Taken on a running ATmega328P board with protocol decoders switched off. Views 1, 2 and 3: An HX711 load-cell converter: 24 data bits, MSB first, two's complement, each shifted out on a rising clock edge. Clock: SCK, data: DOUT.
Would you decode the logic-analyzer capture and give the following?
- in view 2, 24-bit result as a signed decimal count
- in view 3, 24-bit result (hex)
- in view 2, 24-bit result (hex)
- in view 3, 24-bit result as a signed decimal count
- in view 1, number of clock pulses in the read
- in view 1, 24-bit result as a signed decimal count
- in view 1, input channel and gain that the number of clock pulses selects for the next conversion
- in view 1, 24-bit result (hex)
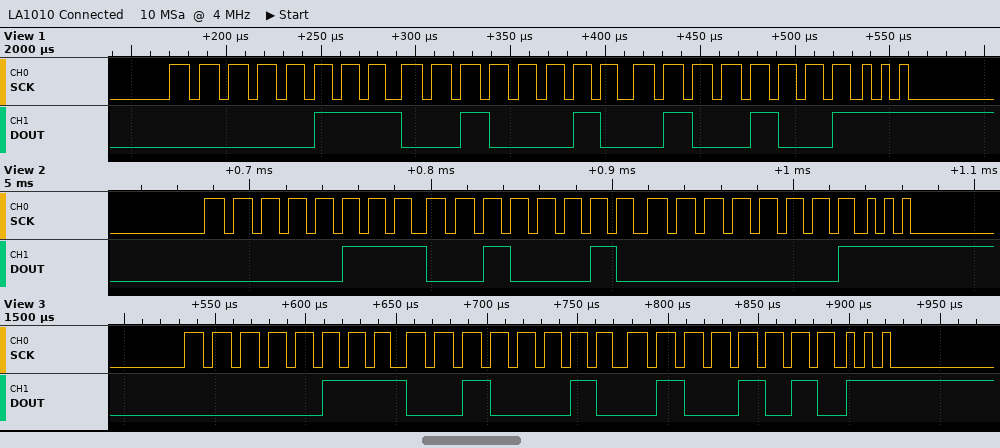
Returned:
467457
0x07224A
0x072201
467530
27
467529
channel A, gain 64
0x072249
